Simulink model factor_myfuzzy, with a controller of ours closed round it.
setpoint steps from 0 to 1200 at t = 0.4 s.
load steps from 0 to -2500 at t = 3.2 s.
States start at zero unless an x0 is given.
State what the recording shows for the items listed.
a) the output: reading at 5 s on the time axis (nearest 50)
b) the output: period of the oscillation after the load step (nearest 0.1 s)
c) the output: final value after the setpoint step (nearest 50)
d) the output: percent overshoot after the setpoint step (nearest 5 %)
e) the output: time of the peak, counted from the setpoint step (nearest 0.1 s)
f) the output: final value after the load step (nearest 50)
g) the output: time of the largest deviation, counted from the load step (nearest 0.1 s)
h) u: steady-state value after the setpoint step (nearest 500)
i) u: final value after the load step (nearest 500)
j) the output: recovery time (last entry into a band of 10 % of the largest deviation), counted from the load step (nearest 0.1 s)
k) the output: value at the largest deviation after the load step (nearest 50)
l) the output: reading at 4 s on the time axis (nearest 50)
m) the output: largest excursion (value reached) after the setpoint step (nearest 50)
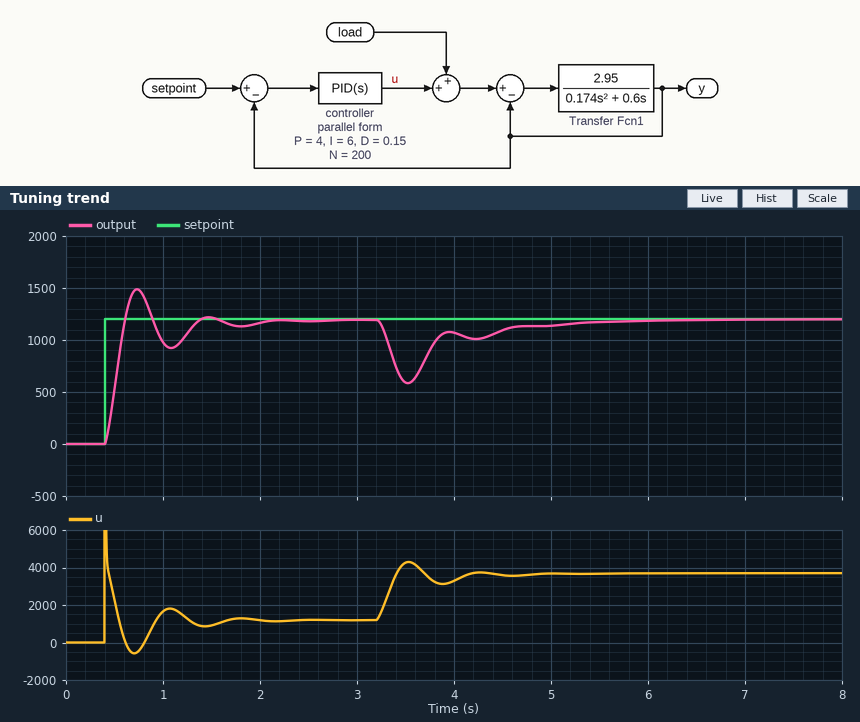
1150
0.7 s
1200
25 %
0.3 s
1200
0.3 s
1000
3500
1.8 s
600
1050
1500
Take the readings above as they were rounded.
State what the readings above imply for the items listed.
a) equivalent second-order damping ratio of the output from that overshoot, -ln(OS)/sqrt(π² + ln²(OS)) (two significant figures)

0.40
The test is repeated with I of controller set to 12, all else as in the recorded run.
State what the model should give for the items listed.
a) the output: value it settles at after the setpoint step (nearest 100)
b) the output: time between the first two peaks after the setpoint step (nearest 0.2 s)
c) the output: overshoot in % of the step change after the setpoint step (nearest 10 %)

1200
0.8 s
40 %
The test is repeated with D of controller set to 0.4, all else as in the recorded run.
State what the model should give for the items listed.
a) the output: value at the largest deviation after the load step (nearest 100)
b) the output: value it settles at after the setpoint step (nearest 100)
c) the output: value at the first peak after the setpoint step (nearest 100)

700
1200
1300
